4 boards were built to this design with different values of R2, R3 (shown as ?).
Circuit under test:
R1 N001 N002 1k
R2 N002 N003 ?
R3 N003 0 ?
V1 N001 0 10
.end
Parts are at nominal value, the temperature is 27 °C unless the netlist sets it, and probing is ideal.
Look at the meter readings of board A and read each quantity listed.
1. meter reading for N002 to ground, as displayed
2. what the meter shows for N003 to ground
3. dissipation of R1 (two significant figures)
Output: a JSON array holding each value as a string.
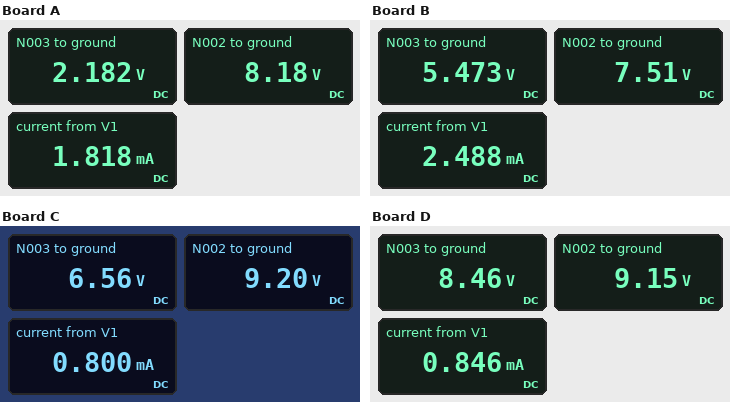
["8.18 V", "2.182 V", "3.3 mW"]
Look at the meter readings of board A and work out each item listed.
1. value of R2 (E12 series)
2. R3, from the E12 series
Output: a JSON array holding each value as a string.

["3.3 kΩ", "1.2 kΩ"]
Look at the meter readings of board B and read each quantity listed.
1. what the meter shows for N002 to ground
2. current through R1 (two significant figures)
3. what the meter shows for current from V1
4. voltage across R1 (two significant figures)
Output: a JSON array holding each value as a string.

["7.51 V", "2.5 mA", "2.488 mA", "2.5 V"]
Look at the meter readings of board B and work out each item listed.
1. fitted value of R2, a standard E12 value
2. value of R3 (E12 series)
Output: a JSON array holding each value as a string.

["820 Ω", "2.2 kΩ"]
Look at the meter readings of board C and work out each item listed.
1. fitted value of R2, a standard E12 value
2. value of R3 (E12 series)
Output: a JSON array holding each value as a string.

["3.3 kΩ", "8.2 kΩ"]
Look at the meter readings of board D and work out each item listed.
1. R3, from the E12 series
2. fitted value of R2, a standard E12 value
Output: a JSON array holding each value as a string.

["10 kΩ", "820 Ω"]
